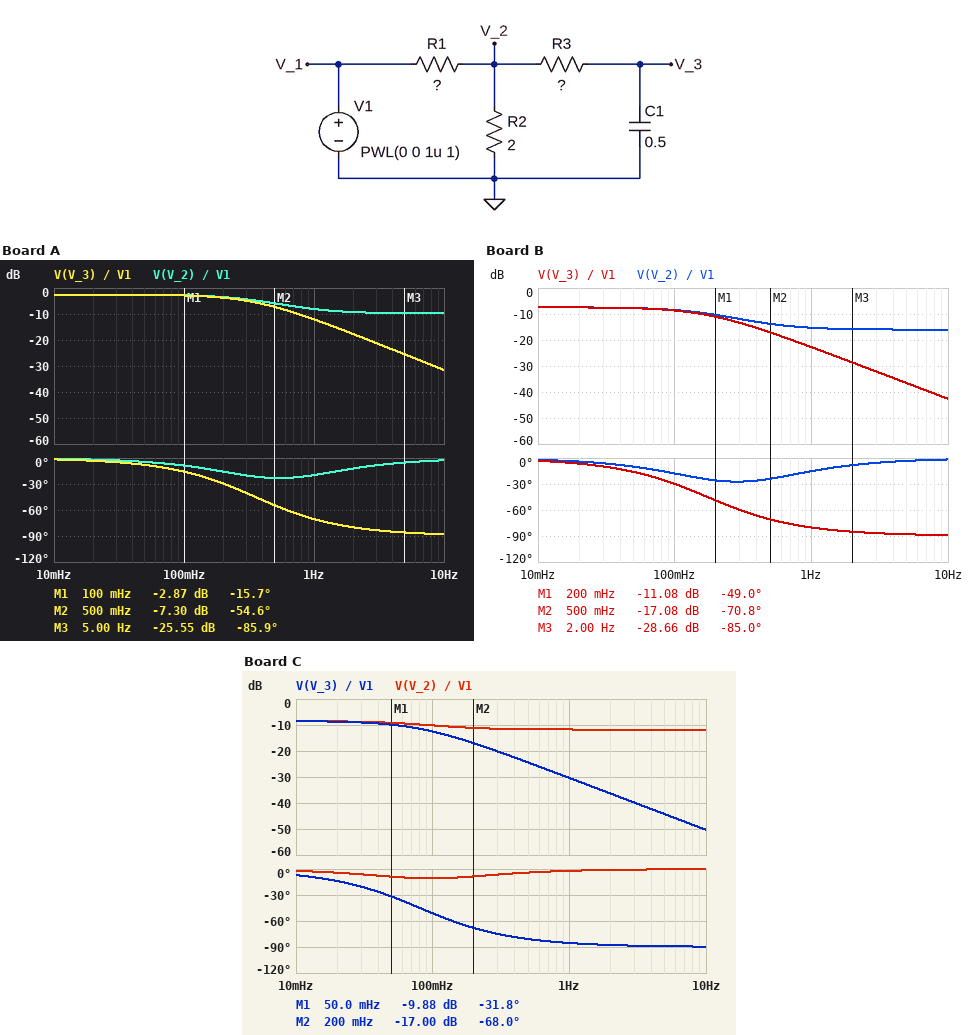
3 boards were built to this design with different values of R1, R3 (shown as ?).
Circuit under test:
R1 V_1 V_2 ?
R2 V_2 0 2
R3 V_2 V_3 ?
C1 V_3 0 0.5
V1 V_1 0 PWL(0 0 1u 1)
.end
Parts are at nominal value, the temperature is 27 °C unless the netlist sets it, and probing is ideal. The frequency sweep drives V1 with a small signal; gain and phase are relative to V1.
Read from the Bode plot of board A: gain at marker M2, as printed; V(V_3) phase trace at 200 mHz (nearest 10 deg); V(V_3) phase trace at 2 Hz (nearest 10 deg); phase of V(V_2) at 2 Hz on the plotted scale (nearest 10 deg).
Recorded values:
-7.30 dB
-30 deg
-80 deg
-10 deg
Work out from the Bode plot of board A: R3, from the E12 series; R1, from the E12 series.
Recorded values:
0.39 Ω
0.68 Ω
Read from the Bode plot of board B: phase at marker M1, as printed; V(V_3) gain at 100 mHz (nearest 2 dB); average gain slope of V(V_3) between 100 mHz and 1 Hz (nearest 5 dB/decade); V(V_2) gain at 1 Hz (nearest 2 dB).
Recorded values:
-49.0 deg
-8 dB
-15 dB/decade
-16 dB
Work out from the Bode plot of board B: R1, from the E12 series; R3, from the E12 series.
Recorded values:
2.7 Ω
0.68 Ω
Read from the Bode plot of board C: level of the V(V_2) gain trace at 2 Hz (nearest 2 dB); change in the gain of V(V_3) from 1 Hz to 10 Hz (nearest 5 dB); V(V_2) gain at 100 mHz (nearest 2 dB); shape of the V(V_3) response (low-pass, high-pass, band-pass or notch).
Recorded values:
-12 dB
-20 dB
-10 dB
low-pass
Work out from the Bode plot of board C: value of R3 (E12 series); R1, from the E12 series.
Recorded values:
2.7 Ω
3.3 Ω
